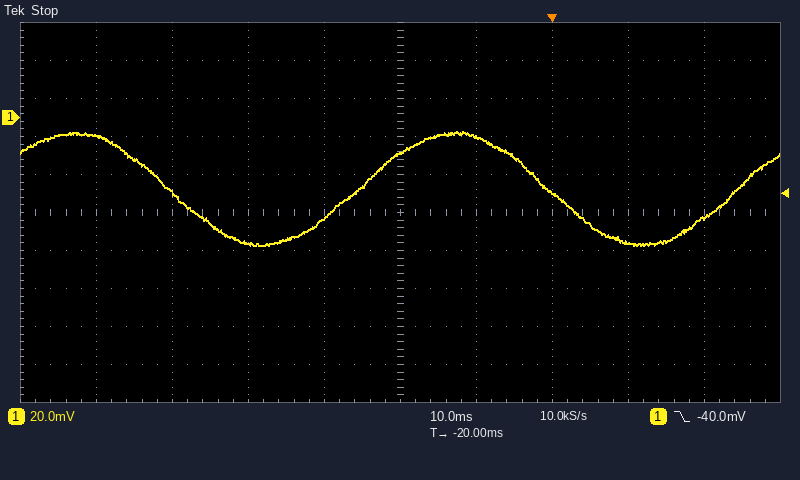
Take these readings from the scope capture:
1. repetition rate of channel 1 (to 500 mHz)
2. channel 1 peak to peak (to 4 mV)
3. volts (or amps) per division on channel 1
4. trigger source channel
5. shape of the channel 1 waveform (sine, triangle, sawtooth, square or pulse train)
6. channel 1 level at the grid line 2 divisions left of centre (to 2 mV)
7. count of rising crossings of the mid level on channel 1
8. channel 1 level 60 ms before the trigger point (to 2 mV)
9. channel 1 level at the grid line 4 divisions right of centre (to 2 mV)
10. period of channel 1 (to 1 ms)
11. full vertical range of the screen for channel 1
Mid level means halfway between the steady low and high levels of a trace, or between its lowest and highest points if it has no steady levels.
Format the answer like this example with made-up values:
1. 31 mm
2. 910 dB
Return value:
1. 20.0 Hz
2. 60 mV
3. 20 mV
4. channel 1
5. sine
6. -66 mV
7. 2
8. -10 mV
9. -52 mV
10. 50 ms
11. 200 mV
